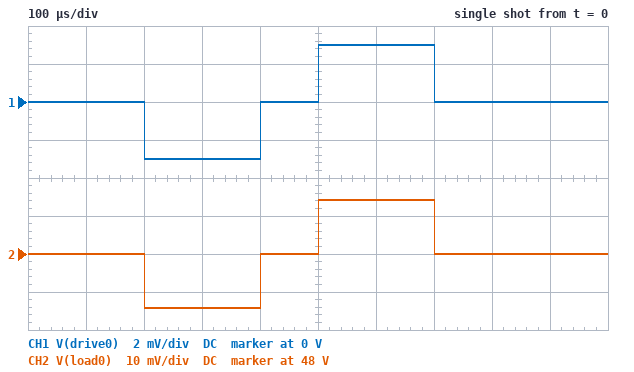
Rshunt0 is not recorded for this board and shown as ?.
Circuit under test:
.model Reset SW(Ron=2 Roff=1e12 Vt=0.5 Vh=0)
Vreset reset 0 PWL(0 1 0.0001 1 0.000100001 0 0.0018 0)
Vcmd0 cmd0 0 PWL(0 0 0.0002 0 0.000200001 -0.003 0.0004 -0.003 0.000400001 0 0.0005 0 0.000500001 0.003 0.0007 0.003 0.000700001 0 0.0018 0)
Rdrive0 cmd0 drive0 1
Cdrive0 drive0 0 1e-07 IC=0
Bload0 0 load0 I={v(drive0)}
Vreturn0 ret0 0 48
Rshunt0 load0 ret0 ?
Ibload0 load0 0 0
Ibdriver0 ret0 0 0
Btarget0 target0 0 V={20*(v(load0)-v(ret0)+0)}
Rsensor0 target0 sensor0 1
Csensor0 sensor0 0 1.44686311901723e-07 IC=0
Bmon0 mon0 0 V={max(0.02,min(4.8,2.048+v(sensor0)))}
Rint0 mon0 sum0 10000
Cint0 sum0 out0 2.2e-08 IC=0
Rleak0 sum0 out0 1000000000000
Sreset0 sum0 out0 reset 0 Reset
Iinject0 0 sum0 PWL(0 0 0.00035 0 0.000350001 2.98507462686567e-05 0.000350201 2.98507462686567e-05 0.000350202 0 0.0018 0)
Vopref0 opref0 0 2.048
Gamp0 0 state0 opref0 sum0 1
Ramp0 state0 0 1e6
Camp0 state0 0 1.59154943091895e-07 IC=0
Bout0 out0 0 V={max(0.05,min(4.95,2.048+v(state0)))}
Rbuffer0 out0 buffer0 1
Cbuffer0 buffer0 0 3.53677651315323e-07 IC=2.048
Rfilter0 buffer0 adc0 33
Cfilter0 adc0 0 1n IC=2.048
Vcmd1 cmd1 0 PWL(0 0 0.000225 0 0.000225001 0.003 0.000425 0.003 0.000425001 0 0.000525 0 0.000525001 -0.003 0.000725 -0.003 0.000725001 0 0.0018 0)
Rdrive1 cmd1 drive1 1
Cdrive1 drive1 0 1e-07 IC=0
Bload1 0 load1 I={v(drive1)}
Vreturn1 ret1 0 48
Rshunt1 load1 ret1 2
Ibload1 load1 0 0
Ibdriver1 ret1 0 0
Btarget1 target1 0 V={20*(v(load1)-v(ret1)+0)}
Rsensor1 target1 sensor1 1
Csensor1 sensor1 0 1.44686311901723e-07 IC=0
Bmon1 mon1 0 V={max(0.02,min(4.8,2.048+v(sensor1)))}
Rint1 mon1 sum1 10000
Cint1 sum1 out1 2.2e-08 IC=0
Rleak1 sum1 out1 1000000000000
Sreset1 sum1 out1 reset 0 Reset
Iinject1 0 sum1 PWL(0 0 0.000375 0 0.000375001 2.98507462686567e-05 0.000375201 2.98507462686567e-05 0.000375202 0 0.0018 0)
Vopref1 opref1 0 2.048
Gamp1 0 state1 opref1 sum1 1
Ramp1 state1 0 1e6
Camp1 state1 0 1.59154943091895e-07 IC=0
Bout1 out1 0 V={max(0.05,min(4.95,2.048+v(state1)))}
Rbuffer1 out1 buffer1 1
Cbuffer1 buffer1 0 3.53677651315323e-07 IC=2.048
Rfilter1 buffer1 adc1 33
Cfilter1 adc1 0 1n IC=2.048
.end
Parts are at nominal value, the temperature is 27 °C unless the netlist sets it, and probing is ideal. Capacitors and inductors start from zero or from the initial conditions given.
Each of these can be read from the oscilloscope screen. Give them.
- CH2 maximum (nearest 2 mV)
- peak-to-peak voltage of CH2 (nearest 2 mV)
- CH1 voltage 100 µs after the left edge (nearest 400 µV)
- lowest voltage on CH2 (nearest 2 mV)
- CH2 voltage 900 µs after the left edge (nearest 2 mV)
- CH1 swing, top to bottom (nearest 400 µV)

48.014 V
28 mV
0 V
47.986 V
48.000 V
6.0 mV
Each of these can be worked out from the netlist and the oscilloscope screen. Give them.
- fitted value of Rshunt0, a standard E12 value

4.7 Ω
